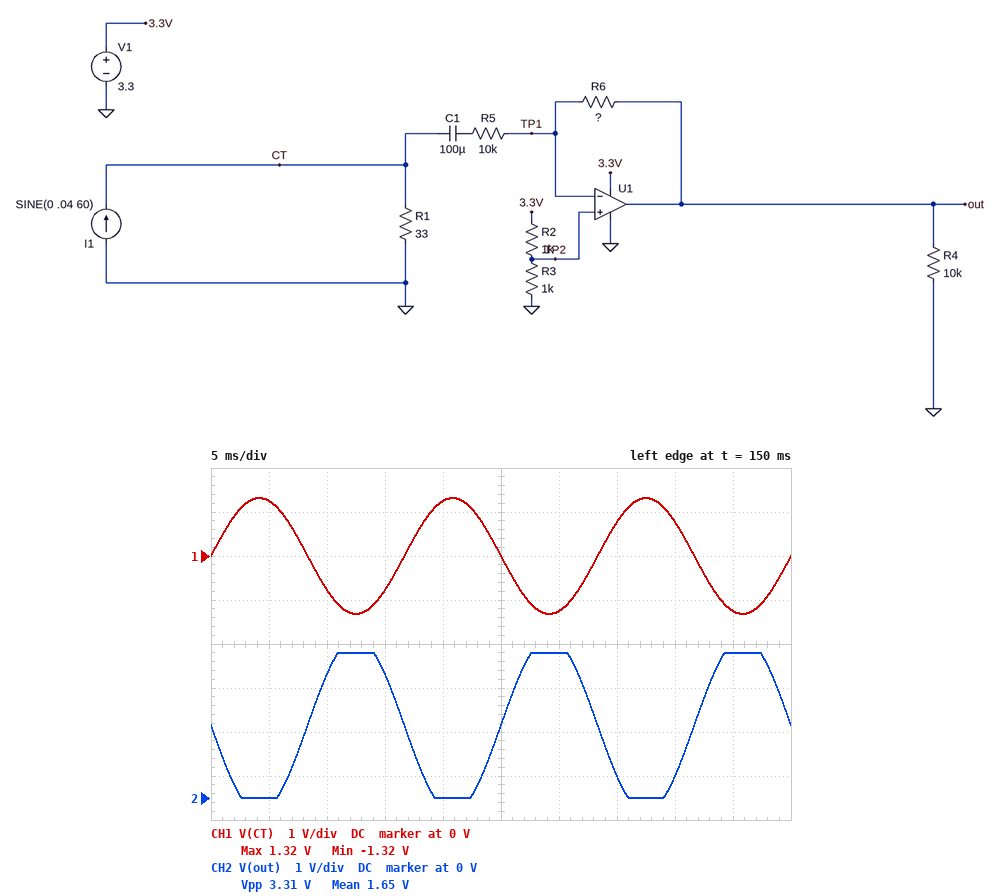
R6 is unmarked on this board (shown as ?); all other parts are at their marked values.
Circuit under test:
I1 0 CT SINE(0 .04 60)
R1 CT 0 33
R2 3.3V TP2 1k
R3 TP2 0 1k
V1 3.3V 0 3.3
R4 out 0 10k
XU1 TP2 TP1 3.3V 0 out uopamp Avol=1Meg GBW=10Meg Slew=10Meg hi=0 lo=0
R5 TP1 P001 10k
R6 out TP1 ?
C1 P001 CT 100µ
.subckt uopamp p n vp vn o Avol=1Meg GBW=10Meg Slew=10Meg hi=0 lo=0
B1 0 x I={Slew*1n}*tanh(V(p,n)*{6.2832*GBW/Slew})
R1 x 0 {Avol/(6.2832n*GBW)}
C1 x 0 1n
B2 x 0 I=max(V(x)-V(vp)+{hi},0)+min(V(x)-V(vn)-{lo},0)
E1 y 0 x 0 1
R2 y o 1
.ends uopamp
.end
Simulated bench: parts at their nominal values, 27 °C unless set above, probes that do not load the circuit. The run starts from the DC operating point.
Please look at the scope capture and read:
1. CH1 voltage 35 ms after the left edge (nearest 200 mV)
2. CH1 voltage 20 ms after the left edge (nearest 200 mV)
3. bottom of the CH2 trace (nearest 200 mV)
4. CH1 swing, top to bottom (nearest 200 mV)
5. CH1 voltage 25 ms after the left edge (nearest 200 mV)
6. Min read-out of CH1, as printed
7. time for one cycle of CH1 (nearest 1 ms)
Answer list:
800 mV
1.2 V
0 V
2.6 V
0 V
-1.32 V
17 ms
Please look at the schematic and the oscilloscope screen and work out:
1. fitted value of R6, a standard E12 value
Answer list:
15 kΩ
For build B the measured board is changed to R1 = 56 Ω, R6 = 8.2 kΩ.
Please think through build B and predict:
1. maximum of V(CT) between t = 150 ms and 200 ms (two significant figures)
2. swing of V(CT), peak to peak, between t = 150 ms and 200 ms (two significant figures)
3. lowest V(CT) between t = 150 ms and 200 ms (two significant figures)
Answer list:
2.2 V
4.5 V
-2.2 V
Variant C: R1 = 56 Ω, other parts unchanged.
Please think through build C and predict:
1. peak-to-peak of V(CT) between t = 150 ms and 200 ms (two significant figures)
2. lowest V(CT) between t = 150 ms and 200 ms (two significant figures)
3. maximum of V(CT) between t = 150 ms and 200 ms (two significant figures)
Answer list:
4.5 V
-2.2 V
2.2 V
